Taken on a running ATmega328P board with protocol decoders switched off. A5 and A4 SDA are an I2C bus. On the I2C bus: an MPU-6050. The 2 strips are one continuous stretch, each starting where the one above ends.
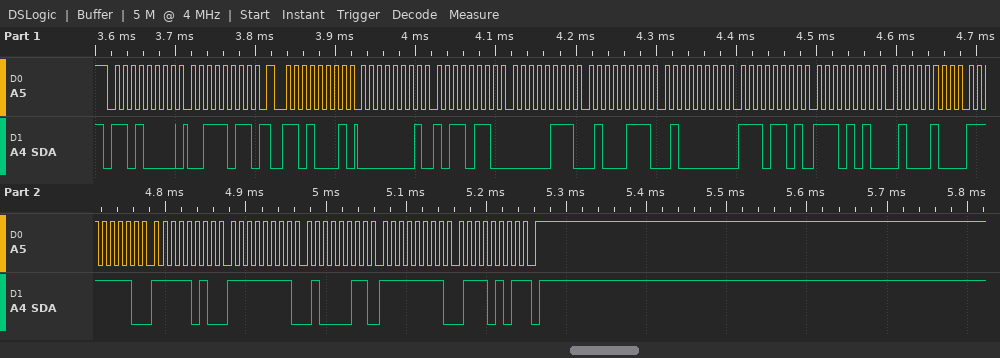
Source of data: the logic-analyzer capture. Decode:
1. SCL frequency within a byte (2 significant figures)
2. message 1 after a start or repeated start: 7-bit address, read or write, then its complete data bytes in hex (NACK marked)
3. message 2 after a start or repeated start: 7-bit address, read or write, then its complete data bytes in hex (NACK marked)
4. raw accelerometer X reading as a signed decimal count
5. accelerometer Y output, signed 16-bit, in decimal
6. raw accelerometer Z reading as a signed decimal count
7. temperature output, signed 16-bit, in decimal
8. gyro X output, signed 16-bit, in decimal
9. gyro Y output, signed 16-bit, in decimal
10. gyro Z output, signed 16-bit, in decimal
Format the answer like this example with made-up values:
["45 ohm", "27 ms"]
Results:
["100 kHz", "0x68 write: 3B", "0x68 read: 01 B6 07 47 40 ED EA 44 FE FA FF 43 FF 75 NACK", "438", "1863", "16621", "-5564", "-262", "-189", "-139"]
